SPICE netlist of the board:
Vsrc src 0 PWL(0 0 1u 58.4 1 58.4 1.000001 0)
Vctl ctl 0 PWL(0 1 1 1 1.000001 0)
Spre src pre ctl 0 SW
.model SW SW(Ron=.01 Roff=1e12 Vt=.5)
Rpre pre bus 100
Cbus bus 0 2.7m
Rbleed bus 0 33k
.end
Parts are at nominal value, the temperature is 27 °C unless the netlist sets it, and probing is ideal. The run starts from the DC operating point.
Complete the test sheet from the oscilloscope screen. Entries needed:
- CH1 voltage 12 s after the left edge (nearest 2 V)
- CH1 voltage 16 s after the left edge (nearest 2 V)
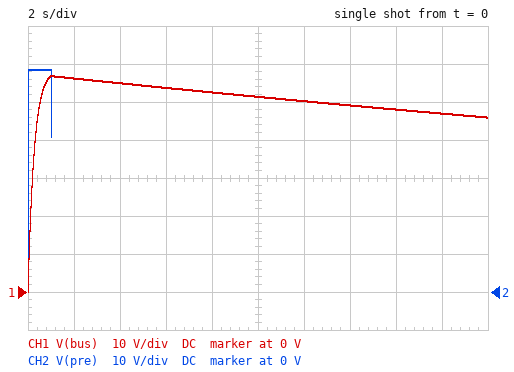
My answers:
50 V
48 V
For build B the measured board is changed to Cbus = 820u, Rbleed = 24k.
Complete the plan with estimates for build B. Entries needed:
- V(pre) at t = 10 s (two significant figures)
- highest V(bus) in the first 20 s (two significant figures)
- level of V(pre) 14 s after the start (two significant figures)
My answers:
37 V
58 V
30 V
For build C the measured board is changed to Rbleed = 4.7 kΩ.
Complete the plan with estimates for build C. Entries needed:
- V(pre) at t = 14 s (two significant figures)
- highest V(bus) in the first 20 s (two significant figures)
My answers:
20 V
56 V
